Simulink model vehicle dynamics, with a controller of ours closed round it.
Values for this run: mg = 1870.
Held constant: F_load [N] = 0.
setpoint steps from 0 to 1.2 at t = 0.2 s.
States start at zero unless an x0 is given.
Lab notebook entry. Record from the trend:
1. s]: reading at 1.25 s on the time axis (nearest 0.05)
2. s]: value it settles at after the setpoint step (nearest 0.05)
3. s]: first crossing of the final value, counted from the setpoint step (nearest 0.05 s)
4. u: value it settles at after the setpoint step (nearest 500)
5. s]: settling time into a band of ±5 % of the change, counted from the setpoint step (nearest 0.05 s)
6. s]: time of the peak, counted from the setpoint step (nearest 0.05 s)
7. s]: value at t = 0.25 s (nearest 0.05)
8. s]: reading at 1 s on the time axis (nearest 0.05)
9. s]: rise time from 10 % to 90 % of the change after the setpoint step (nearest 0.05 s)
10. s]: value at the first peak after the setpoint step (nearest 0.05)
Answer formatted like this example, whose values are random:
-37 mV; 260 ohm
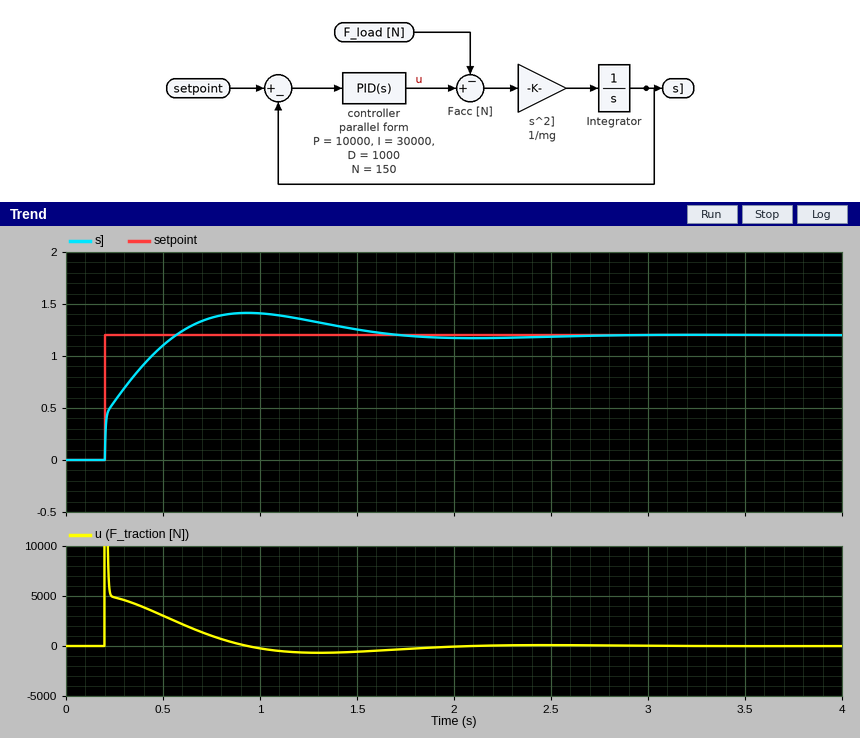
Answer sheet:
1.35; 1.20; 0.35 s; 0; 1.30 s; 0.75 s; 0.55; 1.40; 0.30 s; 1.40
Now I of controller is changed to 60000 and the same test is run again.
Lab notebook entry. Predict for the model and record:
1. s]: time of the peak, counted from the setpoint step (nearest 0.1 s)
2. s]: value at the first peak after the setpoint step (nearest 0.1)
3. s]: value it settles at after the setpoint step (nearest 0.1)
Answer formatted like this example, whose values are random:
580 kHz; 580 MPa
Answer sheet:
0.6 s; 1.5; 1.2
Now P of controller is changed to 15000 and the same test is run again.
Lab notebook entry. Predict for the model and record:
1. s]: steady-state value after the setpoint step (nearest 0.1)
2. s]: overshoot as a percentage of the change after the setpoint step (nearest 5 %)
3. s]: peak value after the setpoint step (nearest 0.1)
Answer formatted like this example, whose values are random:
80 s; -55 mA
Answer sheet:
1.2; 10 %; 1.3
